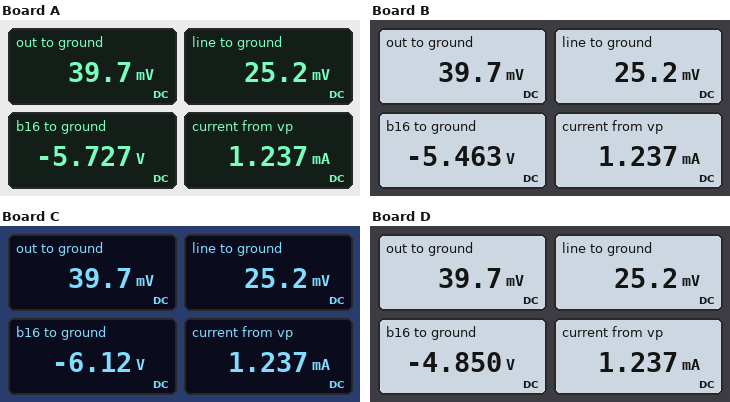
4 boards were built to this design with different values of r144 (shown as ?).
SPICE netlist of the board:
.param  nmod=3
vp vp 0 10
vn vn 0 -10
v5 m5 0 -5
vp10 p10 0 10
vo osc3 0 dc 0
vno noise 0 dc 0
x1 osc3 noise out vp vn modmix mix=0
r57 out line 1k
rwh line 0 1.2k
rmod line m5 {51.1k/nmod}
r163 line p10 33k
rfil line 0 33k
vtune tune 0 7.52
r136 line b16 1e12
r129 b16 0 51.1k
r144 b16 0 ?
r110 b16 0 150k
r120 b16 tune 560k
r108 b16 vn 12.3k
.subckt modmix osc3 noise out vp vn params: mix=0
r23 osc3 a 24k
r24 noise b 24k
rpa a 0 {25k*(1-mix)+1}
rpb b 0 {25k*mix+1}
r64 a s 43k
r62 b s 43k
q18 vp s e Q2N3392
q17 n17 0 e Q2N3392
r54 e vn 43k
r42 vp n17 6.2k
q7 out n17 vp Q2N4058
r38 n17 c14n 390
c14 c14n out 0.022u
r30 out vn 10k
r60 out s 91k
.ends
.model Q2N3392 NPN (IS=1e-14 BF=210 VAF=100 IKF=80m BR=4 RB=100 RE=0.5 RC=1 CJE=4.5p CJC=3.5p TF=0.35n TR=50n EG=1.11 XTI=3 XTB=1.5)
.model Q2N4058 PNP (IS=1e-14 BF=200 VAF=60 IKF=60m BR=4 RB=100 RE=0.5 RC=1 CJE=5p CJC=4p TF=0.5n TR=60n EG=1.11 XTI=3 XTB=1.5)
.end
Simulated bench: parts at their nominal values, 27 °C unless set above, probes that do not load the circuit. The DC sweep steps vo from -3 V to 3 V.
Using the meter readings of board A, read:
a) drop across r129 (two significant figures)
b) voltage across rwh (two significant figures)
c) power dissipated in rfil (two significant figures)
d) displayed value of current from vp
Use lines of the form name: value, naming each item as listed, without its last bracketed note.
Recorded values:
drop across r129: 5.7 V
voltage across rwh: 25 mV
power dissipated in rfil: 19 nW
displayed value of current from vp: 1.237 mA
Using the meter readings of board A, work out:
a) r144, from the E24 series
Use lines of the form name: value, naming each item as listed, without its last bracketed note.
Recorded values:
r144, from the E24 series: 33 kΩ
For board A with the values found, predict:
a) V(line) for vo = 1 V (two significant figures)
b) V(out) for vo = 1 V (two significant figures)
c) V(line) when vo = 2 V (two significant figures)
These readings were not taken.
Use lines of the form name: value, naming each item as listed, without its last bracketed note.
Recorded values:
V(line) for vo = 1 V: -400 mV
V(out) for vo = 1 V: -790 mV
V(line) when vo = 2 V: -810 mV
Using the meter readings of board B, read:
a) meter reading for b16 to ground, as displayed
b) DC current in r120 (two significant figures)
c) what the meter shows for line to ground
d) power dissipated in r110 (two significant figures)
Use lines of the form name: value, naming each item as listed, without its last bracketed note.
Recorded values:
meter reading for b16 to ground, as displayed: -5.463 V
DC current in r120: 23 µA
what the meter shows for line to ground: 25.2 mV
power dissipated in r110: 200 µW
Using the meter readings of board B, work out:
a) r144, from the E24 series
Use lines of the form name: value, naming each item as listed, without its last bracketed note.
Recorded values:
r144, from the E24 series: 27 kΩ
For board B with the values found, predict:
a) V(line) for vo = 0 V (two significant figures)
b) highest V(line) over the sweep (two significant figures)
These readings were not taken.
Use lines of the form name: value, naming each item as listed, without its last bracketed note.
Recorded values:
V(line) for vo = 0 V: 25 mV
highest V(line) over the sweep: 1.3 V
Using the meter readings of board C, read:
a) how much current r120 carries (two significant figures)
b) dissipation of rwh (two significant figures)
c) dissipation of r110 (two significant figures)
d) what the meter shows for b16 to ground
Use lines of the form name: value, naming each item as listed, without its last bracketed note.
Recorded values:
how much current r120 carries: 24 µA
dissipation of rwh: 530 nW
dissipation of r110: 250 µW
what the meter shows for b16 to ground: -6.12 V
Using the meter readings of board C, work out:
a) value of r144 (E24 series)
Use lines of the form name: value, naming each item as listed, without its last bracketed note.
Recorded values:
value of r144: 47 kΩ
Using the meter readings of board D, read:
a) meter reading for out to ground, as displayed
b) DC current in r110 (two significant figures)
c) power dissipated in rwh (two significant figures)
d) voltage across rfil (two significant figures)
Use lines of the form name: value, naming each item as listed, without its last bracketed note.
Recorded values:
meter reading for out to ground, as displayed: 39.7 mV
DC current in r110: 32 µA
power dissipated in rwh: 530 nW
voltage across rfil: 25 mV
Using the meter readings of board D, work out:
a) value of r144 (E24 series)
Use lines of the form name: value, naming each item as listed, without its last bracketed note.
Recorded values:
value of r144: 18 kΩ
